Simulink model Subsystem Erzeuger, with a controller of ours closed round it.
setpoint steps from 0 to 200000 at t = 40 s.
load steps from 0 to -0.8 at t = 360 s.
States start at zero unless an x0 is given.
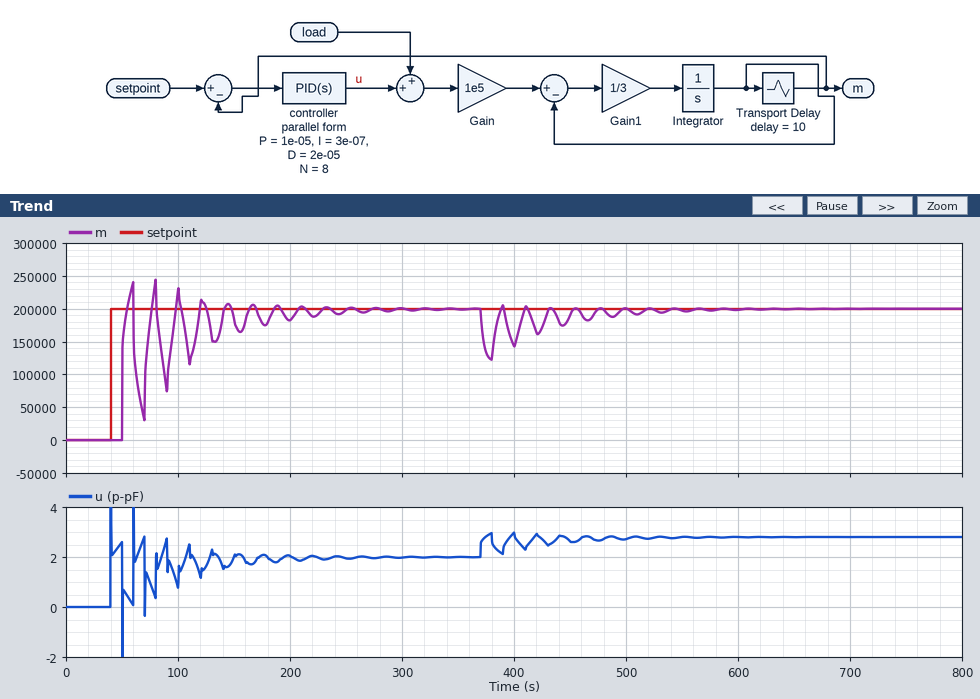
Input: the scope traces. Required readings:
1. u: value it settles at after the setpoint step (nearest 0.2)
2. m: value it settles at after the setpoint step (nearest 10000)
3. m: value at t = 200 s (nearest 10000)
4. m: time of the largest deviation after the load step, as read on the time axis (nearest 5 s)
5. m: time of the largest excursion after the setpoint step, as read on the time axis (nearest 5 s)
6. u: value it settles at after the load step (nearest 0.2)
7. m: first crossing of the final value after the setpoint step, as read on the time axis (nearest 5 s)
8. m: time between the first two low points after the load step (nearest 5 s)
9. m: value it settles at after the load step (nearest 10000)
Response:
2.0
200000
180000
380 s
80 s
2.8
55 s
20 s
200000
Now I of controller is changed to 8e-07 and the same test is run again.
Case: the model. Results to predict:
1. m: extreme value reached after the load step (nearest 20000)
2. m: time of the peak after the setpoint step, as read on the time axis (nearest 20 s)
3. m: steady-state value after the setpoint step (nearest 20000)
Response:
120000
60 s
200000
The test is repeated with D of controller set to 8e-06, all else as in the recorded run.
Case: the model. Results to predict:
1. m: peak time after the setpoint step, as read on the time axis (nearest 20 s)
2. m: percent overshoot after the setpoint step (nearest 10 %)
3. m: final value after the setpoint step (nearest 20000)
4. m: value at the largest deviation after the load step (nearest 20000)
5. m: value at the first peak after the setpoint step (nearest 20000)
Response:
60 s
20 %
200000
120000
240000
